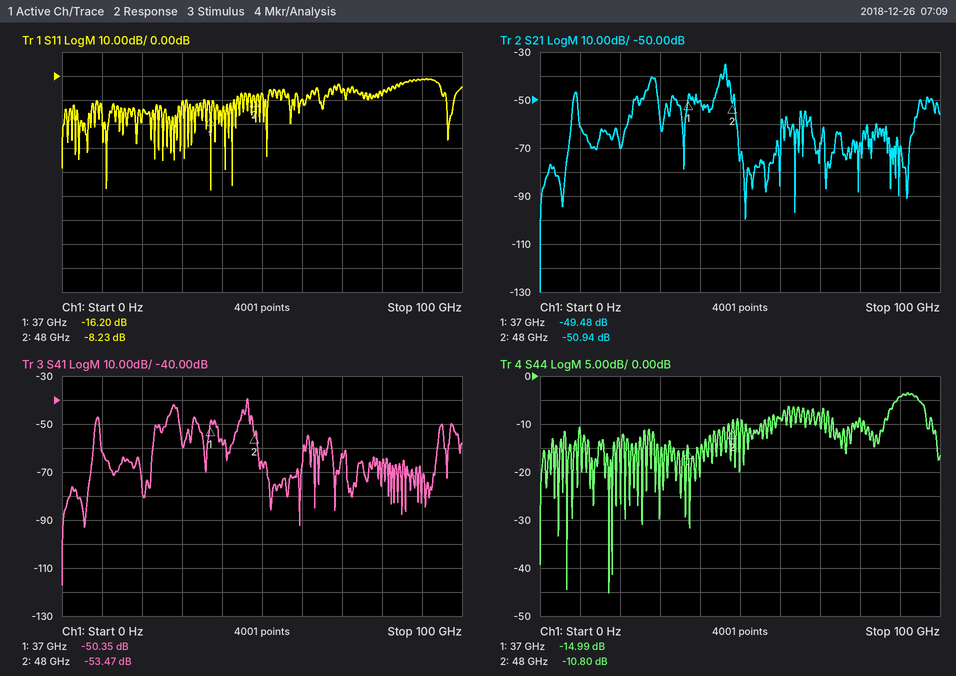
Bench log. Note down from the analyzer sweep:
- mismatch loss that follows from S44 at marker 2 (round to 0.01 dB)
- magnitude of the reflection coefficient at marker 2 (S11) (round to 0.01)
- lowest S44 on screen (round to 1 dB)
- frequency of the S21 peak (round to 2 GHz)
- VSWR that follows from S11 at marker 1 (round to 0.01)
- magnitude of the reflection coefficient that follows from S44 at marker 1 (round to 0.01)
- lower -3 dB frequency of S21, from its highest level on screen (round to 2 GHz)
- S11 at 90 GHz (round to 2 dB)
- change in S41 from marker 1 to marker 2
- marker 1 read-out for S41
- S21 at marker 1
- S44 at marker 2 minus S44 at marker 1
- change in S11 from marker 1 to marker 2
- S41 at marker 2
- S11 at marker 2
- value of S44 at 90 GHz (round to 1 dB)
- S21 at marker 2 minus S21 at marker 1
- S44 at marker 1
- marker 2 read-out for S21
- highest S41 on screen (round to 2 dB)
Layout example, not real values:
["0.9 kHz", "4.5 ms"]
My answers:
["0.38 dB", "0.39", "-45 dB", "46 GHz", "1.37", "0.18", "46 GHz", "-2 dB", "-3.12 dB", "-50.35 dB", "-49.48 dB", "4.19 dB", "7.97 dB", "-53.47 dB", "-8.23 dB", "-4 dB", "-1.46 dB", "-14.99 dB", "-50.94 dB", "-40 dB"]
